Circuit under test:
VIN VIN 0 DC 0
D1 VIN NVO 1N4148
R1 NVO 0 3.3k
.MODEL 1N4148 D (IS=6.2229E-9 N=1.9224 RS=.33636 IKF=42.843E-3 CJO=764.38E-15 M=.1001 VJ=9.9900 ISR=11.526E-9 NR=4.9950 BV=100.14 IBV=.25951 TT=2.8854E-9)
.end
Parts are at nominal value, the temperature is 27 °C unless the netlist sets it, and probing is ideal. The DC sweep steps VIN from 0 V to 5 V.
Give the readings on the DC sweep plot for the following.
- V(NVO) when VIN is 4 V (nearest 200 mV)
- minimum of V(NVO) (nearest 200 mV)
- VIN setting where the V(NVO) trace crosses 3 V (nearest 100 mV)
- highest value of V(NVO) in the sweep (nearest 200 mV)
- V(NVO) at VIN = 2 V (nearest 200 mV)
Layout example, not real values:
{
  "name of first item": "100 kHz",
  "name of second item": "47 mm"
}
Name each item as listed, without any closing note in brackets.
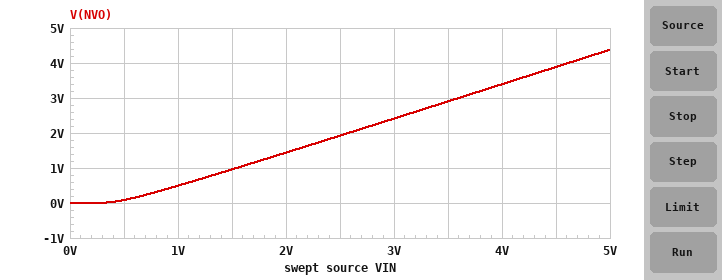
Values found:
{
  "V(NVO) when VIN is 4 V": "3.4 V",
  "minimum of V(NVO)": "0 V",
  "VIN setting where the V(NVO) trace crosses 3 V": "3.6 V",
  "highest value of V(NVO) in the sweep": "4.4 V",
  "V(NVO) at VIN = 2 V": "1.4 V"
}
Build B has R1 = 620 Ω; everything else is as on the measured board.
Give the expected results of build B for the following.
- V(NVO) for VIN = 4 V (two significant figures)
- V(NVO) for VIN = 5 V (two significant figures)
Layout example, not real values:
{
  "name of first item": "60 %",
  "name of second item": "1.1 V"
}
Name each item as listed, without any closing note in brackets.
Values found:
{
  "V(NVO) for VIN = 4 V": "3.3 V",
  "V(NVO) for VIN = 5 V": "4.3 V"
}
